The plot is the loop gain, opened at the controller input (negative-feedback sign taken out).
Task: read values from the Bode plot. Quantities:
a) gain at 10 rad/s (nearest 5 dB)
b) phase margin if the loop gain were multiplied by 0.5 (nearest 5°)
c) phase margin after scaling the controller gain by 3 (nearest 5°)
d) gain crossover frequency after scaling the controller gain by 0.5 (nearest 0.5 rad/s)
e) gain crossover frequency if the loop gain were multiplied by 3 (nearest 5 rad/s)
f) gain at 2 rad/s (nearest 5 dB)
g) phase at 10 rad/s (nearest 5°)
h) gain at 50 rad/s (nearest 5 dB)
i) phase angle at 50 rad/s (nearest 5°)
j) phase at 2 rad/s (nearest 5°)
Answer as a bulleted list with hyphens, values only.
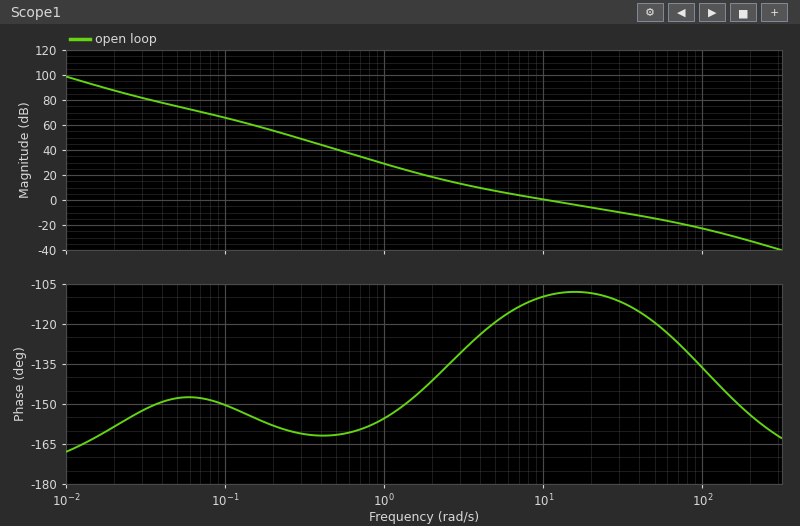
- 0 dB
- 65°
- 70°
- 5.5 rad/s
- 30 rad/s
- 20 dB
- -110°
- -15 dB
- -120°
- -140°
